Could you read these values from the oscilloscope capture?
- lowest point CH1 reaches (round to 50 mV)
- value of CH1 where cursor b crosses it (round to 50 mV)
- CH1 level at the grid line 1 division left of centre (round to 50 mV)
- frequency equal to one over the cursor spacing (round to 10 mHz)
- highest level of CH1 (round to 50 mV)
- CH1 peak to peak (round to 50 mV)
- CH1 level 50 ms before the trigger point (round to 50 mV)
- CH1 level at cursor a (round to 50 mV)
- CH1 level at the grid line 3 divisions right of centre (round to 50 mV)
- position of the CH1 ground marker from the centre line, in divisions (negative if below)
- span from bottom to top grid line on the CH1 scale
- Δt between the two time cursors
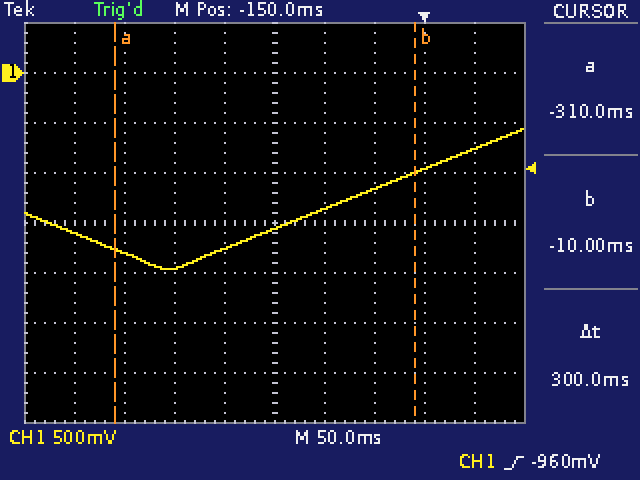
-1.95 V
-1.00 V
-1.75 V
3.33 Hz
-550 mV
1.40 V
-1.15 V
-1.75 V
-950 mV
+3.0 div
4 V
300 ms
